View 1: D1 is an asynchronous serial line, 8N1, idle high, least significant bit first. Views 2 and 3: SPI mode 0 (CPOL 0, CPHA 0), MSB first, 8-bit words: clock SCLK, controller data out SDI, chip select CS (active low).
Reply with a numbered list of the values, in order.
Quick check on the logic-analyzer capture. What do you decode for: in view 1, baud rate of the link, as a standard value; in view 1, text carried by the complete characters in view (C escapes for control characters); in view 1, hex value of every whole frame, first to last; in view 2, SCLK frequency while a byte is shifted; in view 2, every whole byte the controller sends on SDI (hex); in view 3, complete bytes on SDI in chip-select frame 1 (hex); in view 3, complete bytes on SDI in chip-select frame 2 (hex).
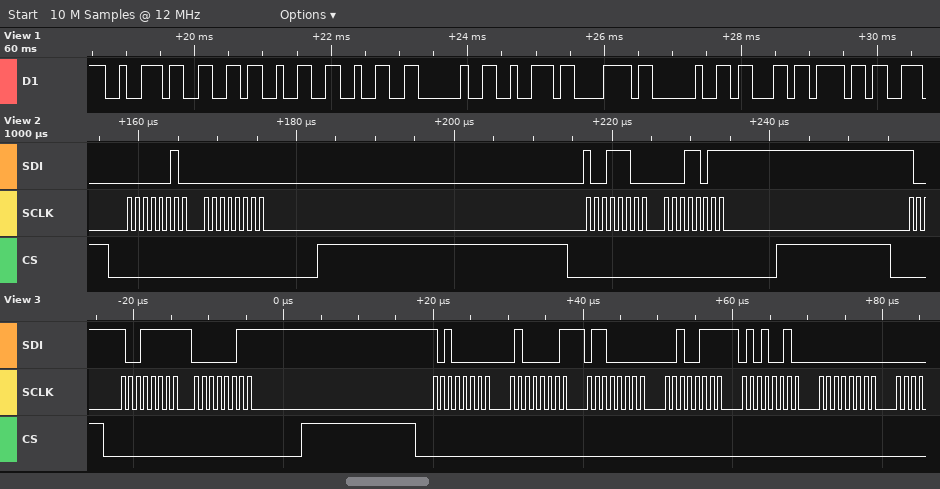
1. 9600 baud
2. "rf22 rx co"
3. 72 66 32 32 20 72 78 20 63 6F
4. 1 MHz
5. 02 00 9C 1B
6. 0x9F 0x03
7. 0xA0 0x41 0x60 0x27 0x52 0x00
